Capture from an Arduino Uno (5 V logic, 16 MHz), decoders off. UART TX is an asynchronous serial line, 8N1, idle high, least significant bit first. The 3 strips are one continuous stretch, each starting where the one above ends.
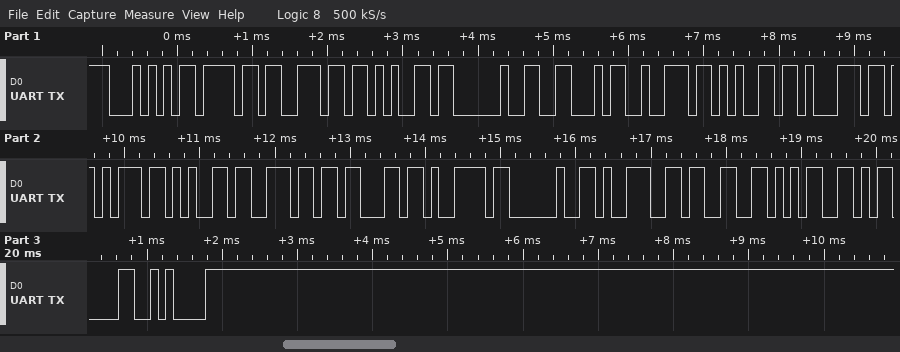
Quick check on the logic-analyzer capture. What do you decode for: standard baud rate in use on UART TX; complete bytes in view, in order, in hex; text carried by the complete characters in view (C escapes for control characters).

9600 baud
0x54 0x6F 0x6E 0x65 0x20 0x46 0x72 0x65 0x71 0x75 0x65 0x6E 0x63 0x79 0x20 0x39 0x33 0x35 0x0D 0x0A
"Tone Frequency 935\r\n"
